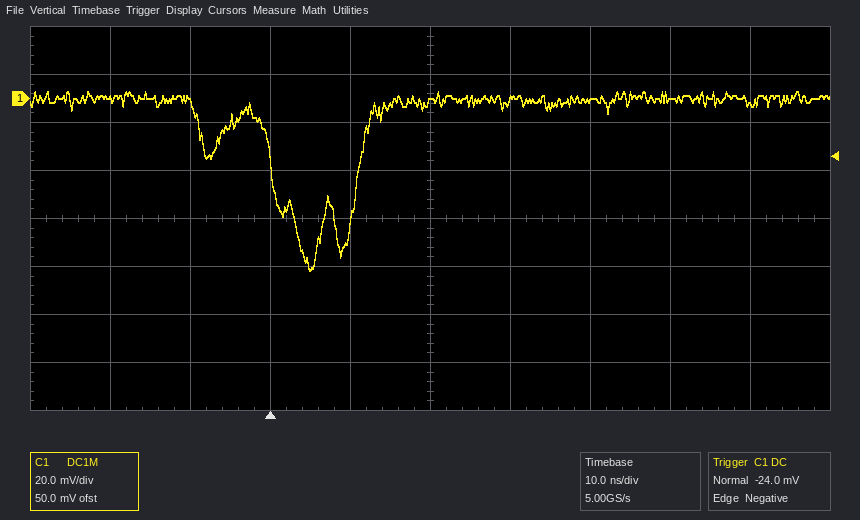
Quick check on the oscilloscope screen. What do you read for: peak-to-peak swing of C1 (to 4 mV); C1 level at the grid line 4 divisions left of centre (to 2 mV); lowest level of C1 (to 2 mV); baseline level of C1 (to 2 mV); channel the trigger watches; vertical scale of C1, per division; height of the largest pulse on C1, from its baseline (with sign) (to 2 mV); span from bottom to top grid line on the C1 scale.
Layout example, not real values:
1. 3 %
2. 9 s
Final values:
1. 76 mV
2. 0 mV
3. -72 mV
4. 0 mV
5. C1
6. 20 mV
7. -72 mV
8. 160 mV
